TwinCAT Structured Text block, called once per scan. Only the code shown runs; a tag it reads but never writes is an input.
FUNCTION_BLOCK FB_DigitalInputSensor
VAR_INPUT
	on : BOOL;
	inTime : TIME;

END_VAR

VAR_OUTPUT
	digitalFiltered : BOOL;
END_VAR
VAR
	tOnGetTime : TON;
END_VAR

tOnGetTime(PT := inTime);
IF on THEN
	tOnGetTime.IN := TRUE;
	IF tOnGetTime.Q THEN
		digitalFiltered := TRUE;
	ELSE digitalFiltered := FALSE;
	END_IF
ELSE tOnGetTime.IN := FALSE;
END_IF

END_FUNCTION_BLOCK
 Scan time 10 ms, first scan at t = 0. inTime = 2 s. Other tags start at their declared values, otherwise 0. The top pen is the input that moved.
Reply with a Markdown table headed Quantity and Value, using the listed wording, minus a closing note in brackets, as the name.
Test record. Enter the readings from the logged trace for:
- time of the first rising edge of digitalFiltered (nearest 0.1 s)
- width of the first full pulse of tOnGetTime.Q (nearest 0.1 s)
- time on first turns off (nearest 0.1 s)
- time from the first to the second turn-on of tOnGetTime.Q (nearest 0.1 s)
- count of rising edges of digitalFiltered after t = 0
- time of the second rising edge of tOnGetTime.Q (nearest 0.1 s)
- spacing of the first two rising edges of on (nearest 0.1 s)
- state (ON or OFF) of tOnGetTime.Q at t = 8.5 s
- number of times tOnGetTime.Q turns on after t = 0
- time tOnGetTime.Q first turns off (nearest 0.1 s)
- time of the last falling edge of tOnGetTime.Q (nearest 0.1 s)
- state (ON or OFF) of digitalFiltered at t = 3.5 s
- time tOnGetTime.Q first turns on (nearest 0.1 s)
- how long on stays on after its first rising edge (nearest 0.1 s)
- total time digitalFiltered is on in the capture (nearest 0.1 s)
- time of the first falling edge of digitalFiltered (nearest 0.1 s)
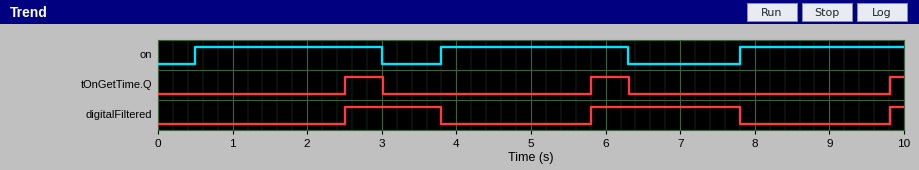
| Quantity | Value |
|---|---|
| time of the first rising edge of digitalFiltered | 2.5 s |
| width of the first full pulse of tOnGetTime.Q | 0.5 s |
| time on first turns off | 3.0 s |
| time from the first to the second turn-on of tOnGetTime.Q | 3.3 s |
| count of rising edges of digitalFiltered after t = 0 | 3 |
| time of the second rising edge of tOnGetTime.Q | 5.8 s |
| spacing of the first two rising edges of on | 3.3 s |
| state (ON or OFF) of tOnGetTime.Q at t = 8.5 s | OFF |
| number of times tOnGetTime.Q turns on after t = 0 | 3 |
| time tOnGetTime.Q first turns off | 3.0 s |
| time of the last falling edge of tOnGetTime.Q | 6.3 s |
| state (ON or OFF) of digitalFiltered at t = 3.5 s | ON |
| time tOnGetTime.Q first turns on | 2.5 s |
| how long on stays on after its first rising edge | 2.5 s |
| total time digitalFiltered is on in the capture | 3.5 s |
| time of the first falling edge of digitalFiltered | 3.8 s |
